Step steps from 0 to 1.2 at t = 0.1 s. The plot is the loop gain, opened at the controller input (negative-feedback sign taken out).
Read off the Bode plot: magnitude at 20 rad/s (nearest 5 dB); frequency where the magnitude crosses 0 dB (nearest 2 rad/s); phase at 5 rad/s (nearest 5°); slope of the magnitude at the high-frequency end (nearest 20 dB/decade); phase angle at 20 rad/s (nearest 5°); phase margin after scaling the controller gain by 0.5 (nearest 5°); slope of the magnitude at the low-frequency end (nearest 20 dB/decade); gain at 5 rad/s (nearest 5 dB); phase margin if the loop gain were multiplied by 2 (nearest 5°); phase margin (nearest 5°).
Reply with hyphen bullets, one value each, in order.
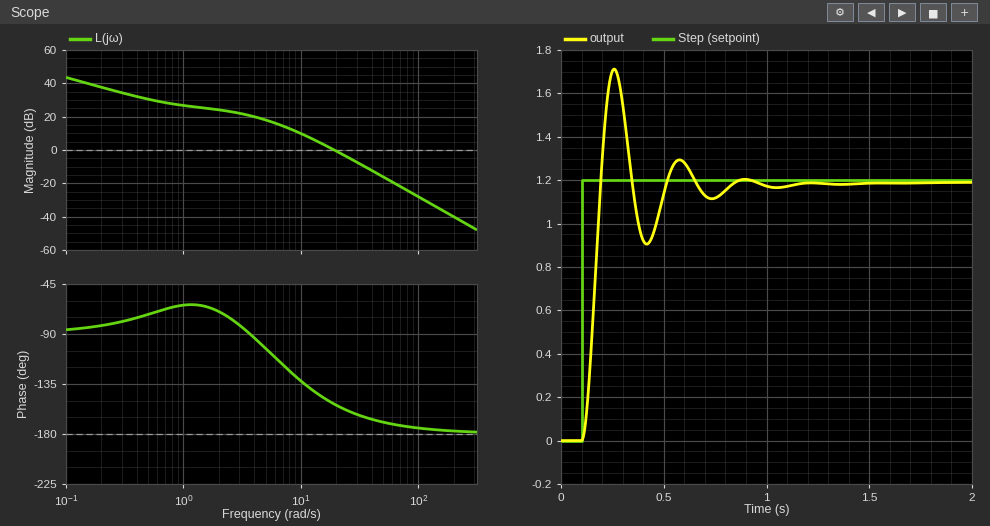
- 0 dB
- 20 rad/s
- -105°
- -40 dB/decade
- -155°
- 40°
- -20 dB/decade
- 20 dB
- 20°
- 25°
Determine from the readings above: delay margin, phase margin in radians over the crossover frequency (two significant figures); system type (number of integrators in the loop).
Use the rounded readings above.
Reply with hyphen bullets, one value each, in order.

- 0.022 s
- 1
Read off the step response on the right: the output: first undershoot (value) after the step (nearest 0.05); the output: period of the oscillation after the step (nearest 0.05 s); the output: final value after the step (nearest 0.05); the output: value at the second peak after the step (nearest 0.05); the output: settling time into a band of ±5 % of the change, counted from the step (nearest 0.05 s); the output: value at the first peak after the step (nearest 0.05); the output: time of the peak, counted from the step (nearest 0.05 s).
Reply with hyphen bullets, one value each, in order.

- 0.90
- 0.30 s
- 1.20
- 1.30
- 0.70 s
- 1.70
- 0.15 s
